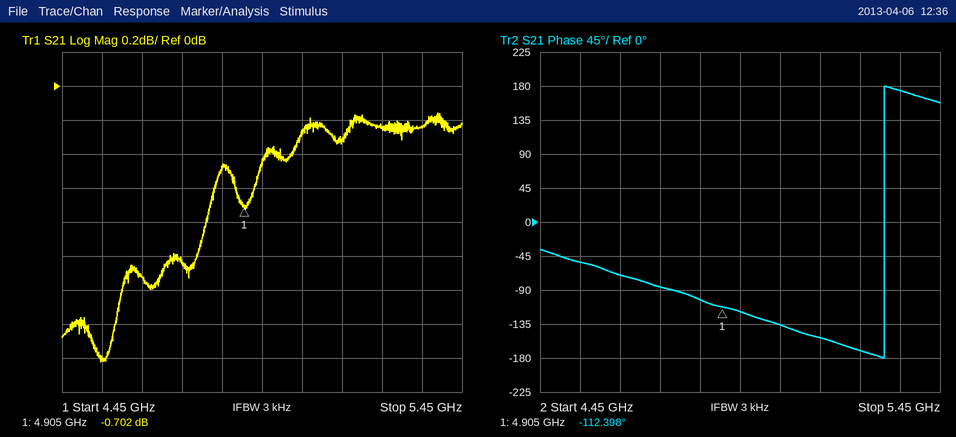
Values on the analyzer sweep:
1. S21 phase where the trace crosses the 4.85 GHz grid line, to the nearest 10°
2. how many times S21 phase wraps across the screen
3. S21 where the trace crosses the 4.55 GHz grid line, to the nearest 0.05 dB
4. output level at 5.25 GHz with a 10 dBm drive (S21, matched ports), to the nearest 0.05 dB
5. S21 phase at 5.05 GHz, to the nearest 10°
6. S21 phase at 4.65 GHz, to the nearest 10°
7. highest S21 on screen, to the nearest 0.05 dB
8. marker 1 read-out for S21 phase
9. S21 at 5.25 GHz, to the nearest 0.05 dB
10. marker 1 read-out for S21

-100°
1
-1.60 dB
9.75 dBm
-140°
-70°
-0.15 dB
-112.398°
-0.25 dB
-0.702 dB
